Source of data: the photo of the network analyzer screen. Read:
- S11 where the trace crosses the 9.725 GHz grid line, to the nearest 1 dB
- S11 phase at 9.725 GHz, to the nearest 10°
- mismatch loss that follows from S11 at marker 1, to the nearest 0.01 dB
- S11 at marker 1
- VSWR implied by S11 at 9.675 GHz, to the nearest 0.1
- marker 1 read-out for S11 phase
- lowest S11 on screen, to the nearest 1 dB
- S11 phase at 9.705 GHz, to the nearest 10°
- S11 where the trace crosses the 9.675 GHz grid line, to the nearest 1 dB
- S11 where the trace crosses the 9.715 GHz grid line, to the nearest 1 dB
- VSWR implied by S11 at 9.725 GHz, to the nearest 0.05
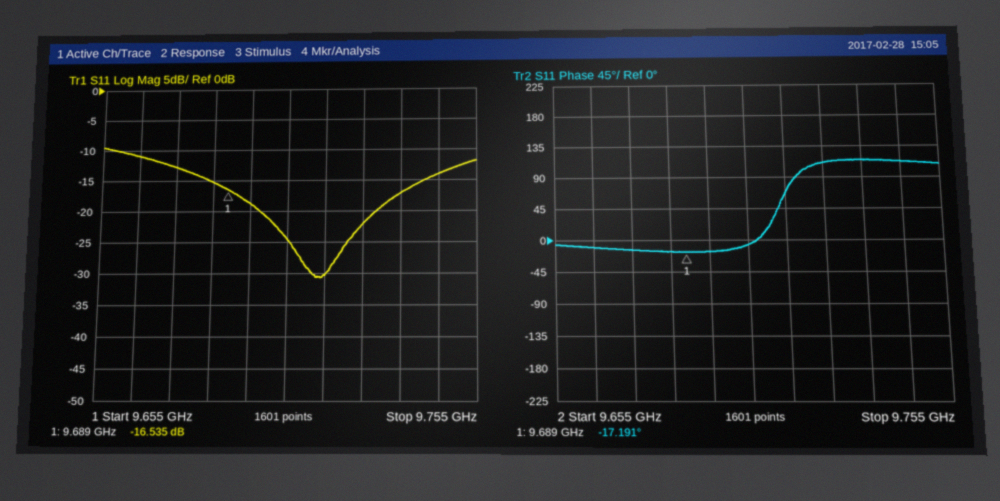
-22 dB
110°
0.10 dB
-16.535 dB
1.6
-17.191°
-31 dB
-10°
-13 dB
-30 dB
1.15
